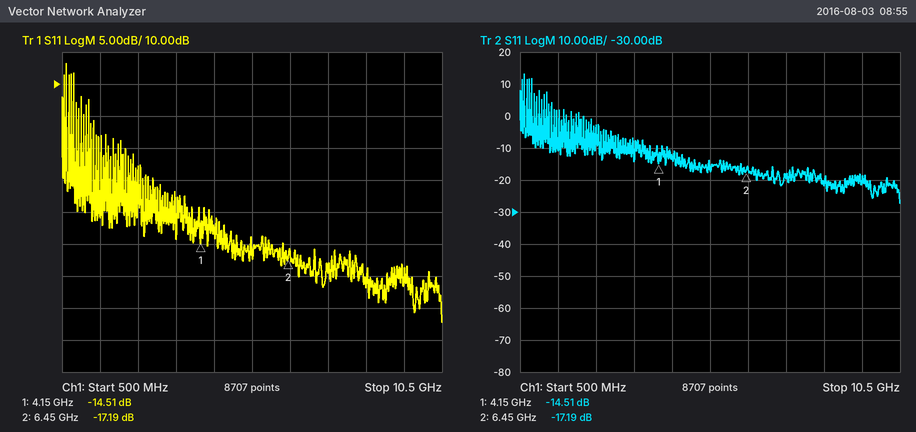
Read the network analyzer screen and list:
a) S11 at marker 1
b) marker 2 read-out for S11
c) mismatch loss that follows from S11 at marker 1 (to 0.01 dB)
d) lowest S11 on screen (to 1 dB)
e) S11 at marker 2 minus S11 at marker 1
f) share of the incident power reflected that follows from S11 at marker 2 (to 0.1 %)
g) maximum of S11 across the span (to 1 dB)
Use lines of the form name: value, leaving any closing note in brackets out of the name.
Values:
S11 at marker 1: -14.51 dB
marker 2 read-out for S11: -17.19 dB
mismatch loss that follows from S11 at marker 1: 0.16 dB
lowest S11 on screen: -27 dB
S11 at marker 2 minus S11 at marker 1: -2.68 dB
share of the incident power reflected that follows from S11 at marker 2: 1.9 %
maximum of S11 across the span: 13 dB
